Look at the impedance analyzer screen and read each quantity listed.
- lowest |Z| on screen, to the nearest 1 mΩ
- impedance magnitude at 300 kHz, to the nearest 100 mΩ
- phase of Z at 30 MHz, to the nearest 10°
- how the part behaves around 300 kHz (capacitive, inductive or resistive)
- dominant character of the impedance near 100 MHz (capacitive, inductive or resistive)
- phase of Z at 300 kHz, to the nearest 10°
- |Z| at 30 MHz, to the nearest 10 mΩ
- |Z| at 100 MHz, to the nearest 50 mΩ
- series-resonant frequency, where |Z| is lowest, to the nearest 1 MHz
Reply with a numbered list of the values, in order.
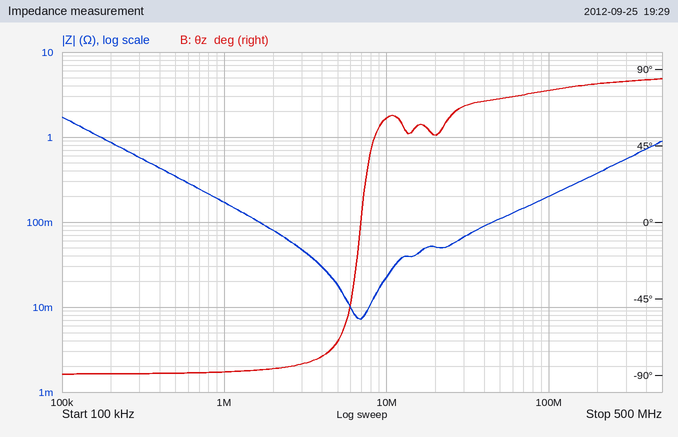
1. 7 mΩ
2. 600 mΩ
3. 70°
4. capacitive
5. inductive
6. -90°
7. 70 mΩ
8. 200 mΩ
9. 7 MHz
